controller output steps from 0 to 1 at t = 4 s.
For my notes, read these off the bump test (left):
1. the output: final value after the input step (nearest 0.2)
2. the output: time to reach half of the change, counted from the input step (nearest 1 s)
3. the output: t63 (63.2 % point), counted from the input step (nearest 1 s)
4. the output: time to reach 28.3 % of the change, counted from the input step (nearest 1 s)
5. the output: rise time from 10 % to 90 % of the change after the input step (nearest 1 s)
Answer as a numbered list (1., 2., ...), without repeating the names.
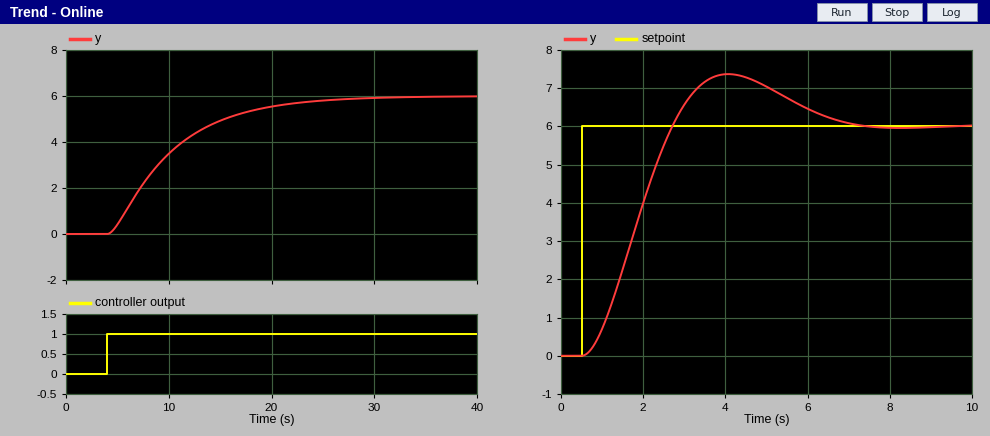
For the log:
1. 6.0
2. 5 s
3. 7 s
4. 3 s
5. 13 s
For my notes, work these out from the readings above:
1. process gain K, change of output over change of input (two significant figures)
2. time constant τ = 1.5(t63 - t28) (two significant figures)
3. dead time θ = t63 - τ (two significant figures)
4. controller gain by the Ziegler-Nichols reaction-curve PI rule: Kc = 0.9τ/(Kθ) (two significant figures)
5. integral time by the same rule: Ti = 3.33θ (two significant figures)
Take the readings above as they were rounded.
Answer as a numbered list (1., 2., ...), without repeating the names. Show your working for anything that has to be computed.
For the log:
1. (6 - 0) / 1 = 6.0
2. 1.5 × (7 - 3) = 6.0 s
3. 7 - 6 = 1.0 s
4. 0.9 × 6 / (6 × 1) = 0.90
5. 3.33 × 1 = 3.3 s
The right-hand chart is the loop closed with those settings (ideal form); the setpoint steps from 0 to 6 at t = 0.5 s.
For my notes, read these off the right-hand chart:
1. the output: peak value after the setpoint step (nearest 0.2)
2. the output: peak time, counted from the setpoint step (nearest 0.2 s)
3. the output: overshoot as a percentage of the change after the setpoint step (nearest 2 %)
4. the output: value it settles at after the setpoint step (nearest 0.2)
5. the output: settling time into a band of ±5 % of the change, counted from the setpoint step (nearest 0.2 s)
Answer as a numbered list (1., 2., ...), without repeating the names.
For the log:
1. 7.4
2. 3.6 s
3. 22 %
4. 6.0
5. 5.8 s
